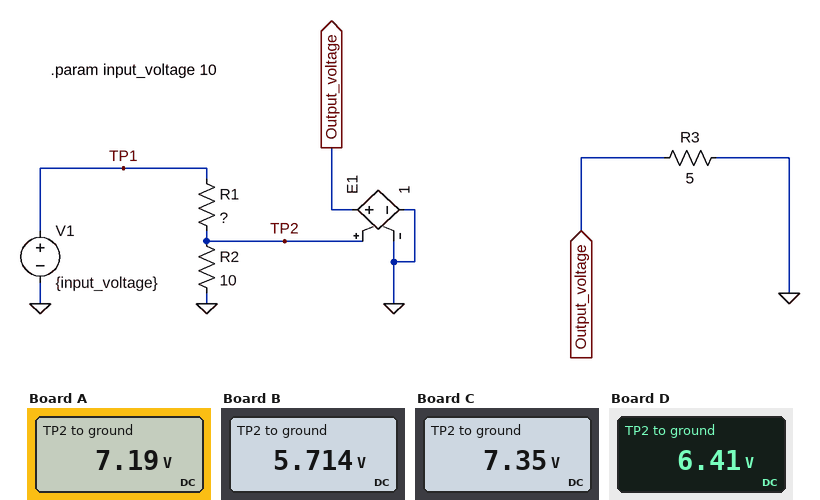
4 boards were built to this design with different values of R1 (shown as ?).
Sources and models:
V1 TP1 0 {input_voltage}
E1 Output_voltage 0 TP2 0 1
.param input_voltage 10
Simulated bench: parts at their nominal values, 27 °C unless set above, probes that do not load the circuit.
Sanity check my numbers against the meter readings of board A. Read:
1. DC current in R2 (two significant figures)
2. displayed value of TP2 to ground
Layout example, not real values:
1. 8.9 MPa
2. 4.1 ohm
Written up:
1. 720 mA
2. 7.19 V
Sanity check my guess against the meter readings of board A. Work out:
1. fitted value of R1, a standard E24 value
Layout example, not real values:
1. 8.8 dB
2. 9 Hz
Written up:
1. 3.9 Ω
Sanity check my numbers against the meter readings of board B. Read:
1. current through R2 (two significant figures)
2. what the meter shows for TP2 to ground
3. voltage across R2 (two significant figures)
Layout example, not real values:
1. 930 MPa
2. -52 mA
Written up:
1. 570 mA
2. 5.714 V
3. 5.7 V
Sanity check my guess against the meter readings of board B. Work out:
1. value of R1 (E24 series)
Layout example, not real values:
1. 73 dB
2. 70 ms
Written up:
1. 7.5 Ω
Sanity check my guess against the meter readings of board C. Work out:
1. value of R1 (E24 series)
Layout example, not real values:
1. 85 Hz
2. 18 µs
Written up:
1. 3.6 Ω
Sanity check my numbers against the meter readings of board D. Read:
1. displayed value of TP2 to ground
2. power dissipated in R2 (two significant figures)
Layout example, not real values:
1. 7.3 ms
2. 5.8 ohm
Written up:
1. 6.41 V
2. 4.1 W
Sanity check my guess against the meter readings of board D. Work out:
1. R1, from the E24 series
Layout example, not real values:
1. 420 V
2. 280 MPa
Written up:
1. 5.6 Ω
